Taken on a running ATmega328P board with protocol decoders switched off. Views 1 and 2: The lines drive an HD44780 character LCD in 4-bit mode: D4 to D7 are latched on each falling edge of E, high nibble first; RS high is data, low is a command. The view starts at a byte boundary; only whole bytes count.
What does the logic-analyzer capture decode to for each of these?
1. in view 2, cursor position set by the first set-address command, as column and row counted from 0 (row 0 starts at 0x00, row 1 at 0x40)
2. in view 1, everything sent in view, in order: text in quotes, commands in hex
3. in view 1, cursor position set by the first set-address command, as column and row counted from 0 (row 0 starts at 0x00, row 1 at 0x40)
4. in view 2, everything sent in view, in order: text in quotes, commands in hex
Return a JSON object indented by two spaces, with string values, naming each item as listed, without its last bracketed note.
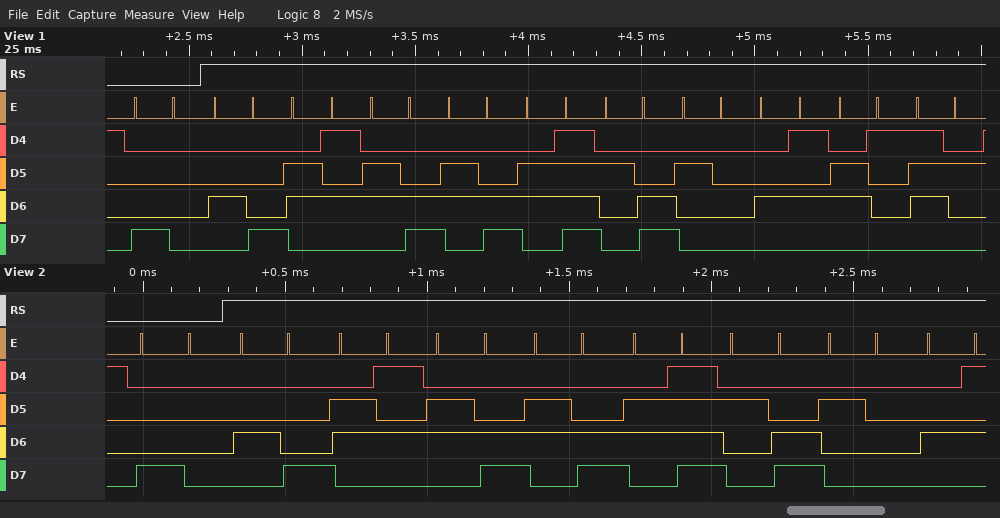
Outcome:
{
  "in view 2, cursor position set by the first set-address command, as column and row counted from 0": "column 0, row 0",
  "in view 1, everything sent in view, in order: text in quotes, commands in hex": "0x80 \"Hello, Ear\"",
  "in view 1, cursor position set by the first set-address command, as column and row counted from 0": "column 0, row 0",
  "in view 2, everything sent in view, in order: text in quotes, commands in hex": "0x80 \"Hello, E\""
}
